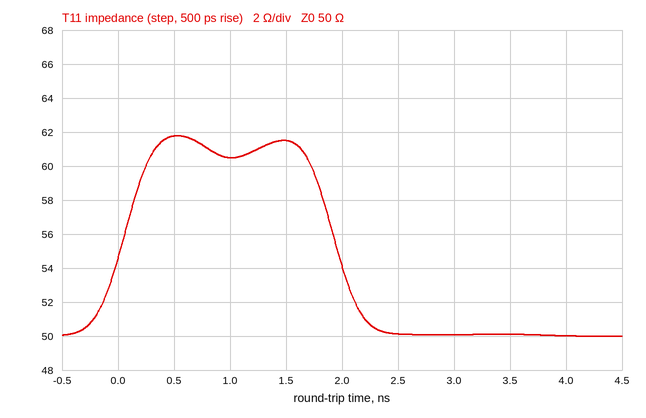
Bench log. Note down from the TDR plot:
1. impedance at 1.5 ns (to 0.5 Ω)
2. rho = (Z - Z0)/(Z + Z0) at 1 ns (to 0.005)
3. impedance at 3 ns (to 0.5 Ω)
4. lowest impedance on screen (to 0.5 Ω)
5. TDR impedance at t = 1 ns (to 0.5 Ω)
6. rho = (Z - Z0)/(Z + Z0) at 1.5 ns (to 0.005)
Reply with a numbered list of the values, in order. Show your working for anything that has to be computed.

1. 61.5 Ω
2. (60.5 − 50)/(60.5 + 50) ≈ +0.095
3. 50.0 Ω
4. 50.0 Ω
5. 60.5 Ω
6. (61.5 − 50)/(61.5 + 50) ≈ +0.103, so +0.105 to the nearest 0.005
